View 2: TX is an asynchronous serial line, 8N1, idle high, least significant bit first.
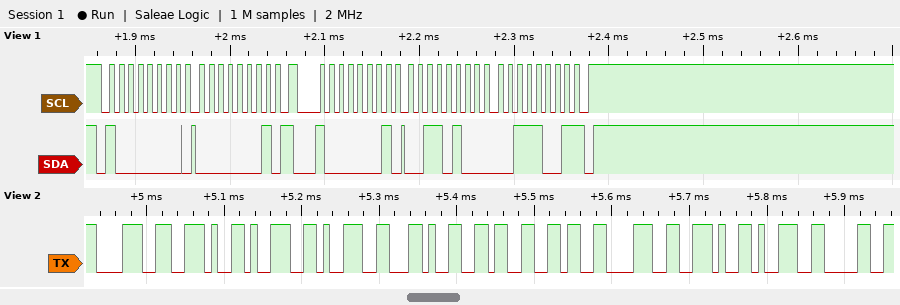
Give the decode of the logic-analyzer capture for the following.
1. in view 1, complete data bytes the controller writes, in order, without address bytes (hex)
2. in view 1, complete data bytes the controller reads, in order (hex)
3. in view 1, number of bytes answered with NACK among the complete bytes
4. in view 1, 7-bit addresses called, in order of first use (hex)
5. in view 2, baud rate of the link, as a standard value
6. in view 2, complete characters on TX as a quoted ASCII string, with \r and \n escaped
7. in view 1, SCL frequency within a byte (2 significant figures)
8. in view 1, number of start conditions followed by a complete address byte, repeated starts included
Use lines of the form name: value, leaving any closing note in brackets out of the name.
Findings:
in view 1, complete data bytes the controller writes, in order, without address bytes: 01
in view 1, complete data bytes the controller reads, in order: 34 39
in view 1, number of bytes answered with NACK among the complete bytes: 1
in view 1, 7-bit addresses called, in order of first use: 0x40
in view 2, baud rate of the link, as a standard value: 115200 baud
in view 2, complete characters on TX as a quoted ASCII string, with \r and \n escaped: "8.99,668.90"
in view 1, SCL frequency within a byte: 100 kHz
in view 1, number of start conditions followed by a complete address byte, repeated starts included: 2
